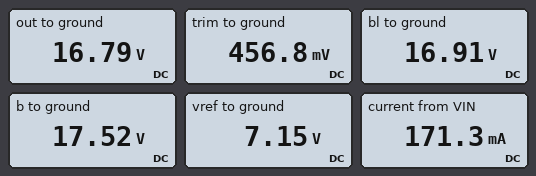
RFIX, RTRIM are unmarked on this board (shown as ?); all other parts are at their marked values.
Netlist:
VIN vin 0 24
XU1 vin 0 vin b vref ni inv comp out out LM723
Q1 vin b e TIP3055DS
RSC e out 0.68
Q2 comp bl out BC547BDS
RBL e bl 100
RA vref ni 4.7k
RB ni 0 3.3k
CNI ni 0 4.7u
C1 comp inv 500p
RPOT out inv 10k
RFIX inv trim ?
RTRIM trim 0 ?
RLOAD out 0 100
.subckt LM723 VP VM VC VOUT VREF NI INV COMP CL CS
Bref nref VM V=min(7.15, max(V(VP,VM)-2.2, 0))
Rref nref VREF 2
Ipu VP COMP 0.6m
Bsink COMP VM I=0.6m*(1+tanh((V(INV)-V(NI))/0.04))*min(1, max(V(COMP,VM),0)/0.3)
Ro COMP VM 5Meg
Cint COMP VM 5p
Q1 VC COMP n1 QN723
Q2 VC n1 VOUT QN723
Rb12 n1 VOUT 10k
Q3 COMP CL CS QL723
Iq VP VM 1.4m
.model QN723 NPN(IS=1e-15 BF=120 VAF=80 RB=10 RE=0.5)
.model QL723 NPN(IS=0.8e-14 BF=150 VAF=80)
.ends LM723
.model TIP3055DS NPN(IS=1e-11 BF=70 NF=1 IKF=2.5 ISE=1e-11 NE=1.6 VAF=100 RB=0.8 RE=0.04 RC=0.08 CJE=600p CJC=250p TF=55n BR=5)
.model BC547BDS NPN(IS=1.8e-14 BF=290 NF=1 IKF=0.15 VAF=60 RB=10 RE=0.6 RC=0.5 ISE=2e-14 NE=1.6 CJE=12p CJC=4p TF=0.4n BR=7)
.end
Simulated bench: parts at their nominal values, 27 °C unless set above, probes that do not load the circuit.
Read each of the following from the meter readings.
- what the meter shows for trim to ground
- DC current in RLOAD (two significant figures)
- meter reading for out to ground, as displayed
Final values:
456.8 mV
170 mA
16.79 V
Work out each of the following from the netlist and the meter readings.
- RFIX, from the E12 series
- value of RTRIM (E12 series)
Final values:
1.8 kΩ
330 Ω
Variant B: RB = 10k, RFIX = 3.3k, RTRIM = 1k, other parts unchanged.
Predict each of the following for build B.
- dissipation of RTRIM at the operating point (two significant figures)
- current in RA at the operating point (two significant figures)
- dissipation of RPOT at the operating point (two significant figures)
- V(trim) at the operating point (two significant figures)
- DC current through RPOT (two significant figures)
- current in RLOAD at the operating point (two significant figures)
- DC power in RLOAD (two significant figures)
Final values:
1.3 mW
490 µA
13 mW
1.1 V
1.1 mA
160 mA
2.6 W
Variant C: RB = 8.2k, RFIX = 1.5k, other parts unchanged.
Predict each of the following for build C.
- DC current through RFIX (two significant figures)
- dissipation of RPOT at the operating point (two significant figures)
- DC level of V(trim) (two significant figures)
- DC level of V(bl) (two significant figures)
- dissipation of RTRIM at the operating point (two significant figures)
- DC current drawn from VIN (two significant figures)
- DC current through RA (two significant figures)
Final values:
1.9 mA
36 mW
630 mV
23 V
1.2 mW
230 mA
550 µA
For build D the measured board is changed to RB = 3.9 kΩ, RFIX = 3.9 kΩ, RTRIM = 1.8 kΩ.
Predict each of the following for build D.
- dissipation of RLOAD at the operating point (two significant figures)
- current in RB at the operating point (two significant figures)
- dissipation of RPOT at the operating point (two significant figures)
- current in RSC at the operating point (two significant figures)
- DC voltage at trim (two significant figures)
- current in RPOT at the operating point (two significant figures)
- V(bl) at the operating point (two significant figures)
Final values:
800 mW
830 µA
3.2 mW
90 mA
1.0 V
570 µA
9.0 V
